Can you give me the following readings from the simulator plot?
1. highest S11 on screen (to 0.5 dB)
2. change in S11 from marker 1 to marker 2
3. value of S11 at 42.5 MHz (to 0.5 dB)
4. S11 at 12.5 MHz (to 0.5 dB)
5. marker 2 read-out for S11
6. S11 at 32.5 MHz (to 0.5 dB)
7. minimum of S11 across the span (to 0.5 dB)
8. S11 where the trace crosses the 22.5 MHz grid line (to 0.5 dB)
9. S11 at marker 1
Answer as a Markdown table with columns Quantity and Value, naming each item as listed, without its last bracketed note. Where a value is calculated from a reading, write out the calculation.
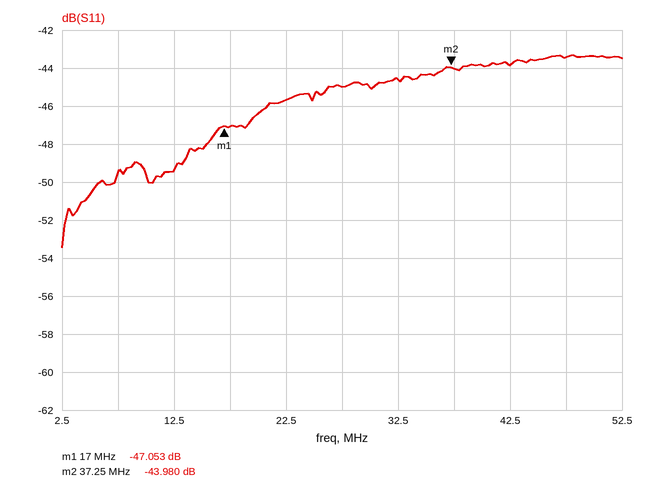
| Quantity | Value |
|---|---|
| highest S11 on screen | -43.5 dB |
| change in S11 from marker 1 to marker 2 | -43.98 − (-47.053) = 3.073 dB |
| value of S11 at 42.5 MHz | -44.0 dB |
| S11 at 12.5 MHz | -49.5 dB |
| marker 2 read-out for S11 | -43.980 dB |
| S11 at 32.5 MHz | -44.5 dB |
| minimum of S11 across the span | -53.5 dB |
| S11 where the trace crosses the 22.5 MHz grid line | -45.5 dB |
| S11 at marker 1 | -47.053 dB |
